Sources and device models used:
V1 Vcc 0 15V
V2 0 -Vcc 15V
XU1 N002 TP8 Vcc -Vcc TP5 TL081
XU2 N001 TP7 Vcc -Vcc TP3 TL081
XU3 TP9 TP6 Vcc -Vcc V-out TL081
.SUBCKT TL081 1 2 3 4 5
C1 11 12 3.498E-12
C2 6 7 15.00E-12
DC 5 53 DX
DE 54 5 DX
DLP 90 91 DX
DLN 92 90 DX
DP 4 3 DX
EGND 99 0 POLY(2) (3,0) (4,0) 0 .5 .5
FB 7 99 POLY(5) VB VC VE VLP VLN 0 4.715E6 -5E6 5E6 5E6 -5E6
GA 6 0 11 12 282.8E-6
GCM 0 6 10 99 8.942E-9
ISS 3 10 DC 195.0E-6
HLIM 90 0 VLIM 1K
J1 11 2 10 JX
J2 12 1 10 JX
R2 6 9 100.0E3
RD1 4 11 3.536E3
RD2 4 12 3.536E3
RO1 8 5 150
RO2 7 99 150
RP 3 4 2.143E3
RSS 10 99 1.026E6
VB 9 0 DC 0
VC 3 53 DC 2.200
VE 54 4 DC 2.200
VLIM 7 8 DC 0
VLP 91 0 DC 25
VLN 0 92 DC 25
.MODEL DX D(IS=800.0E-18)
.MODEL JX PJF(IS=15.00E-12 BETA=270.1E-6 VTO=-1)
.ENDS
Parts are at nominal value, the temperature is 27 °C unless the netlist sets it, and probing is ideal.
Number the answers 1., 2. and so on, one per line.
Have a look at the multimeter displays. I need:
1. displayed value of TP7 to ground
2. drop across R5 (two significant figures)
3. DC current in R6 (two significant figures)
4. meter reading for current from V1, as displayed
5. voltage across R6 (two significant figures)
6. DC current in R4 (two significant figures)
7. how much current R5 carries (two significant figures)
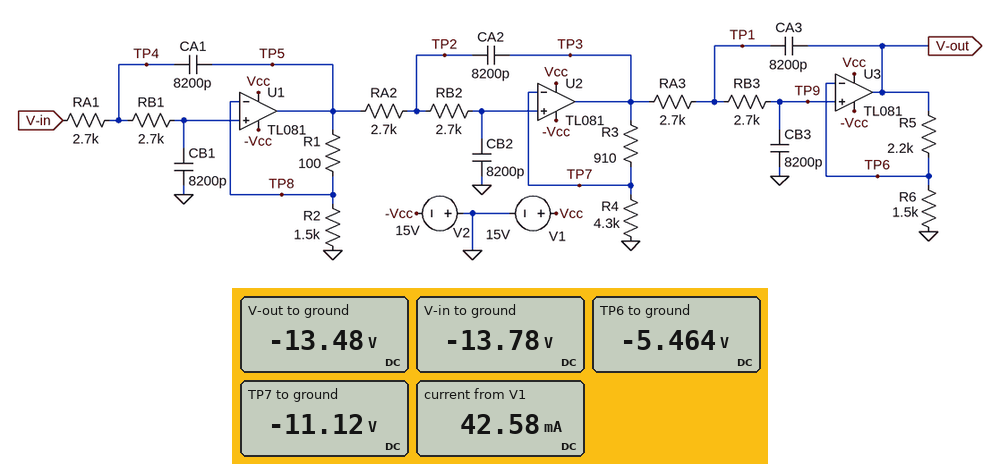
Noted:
1. -11.12 V
2. 8.0 V
3. 3.6 mA
4. 42.58 mA
5. 5.5 V
6. 2.6 mA
7. 3.6 mA
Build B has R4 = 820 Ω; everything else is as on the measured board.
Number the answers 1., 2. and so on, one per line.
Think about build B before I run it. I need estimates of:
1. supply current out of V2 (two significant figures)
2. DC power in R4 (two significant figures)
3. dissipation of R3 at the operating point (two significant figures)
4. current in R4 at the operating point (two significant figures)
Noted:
1. 42 mA
2. 50 mW
3. 55 mW
4. 7.8 mA
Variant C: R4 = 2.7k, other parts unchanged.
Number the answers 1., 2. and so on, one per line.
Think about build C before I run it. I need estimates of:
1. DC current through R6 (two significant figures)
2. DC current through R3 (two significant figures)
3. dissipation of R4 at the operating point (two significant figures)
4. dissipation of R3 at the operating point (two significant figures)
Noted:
1. 3.6 mA
2. 3.7 mA
3. 38 mW
4. 13 mW
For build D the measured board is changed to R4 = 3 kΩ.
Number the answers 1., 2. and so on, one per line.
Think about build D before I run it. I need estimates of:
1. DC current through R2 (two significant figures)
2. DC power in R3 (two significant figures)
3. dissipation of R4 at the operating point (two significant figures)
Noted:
1. 8.4 mA
2. 11 mW
3. 36 mW
